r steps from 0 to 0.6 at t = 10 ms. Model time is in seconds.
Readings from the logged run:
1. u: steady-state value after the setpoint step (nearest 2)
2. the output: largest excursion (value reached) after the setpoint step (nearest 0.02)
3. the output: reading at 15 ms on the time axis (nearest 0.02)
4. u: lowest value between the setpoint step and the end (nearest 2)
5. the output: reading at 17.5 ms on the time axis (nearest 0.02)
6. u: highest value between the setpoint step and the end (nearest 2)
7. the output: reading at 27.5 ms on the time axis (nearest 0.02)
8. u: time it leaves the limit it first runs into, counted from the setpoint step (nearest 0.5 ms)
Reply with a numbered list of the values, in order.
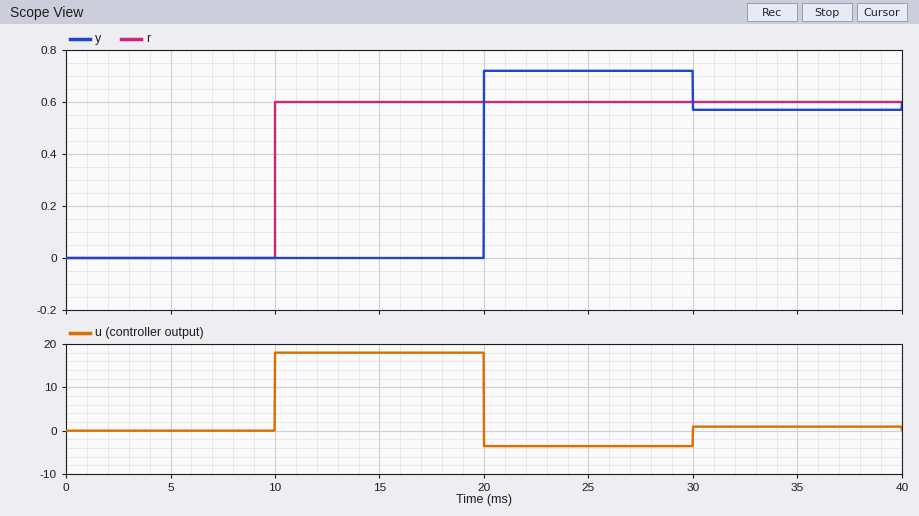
1. 0
2. 0.72
3. 0.00
4. -4
5. 0.00
6. 18
7. 0.72
8. 10.0 ms
